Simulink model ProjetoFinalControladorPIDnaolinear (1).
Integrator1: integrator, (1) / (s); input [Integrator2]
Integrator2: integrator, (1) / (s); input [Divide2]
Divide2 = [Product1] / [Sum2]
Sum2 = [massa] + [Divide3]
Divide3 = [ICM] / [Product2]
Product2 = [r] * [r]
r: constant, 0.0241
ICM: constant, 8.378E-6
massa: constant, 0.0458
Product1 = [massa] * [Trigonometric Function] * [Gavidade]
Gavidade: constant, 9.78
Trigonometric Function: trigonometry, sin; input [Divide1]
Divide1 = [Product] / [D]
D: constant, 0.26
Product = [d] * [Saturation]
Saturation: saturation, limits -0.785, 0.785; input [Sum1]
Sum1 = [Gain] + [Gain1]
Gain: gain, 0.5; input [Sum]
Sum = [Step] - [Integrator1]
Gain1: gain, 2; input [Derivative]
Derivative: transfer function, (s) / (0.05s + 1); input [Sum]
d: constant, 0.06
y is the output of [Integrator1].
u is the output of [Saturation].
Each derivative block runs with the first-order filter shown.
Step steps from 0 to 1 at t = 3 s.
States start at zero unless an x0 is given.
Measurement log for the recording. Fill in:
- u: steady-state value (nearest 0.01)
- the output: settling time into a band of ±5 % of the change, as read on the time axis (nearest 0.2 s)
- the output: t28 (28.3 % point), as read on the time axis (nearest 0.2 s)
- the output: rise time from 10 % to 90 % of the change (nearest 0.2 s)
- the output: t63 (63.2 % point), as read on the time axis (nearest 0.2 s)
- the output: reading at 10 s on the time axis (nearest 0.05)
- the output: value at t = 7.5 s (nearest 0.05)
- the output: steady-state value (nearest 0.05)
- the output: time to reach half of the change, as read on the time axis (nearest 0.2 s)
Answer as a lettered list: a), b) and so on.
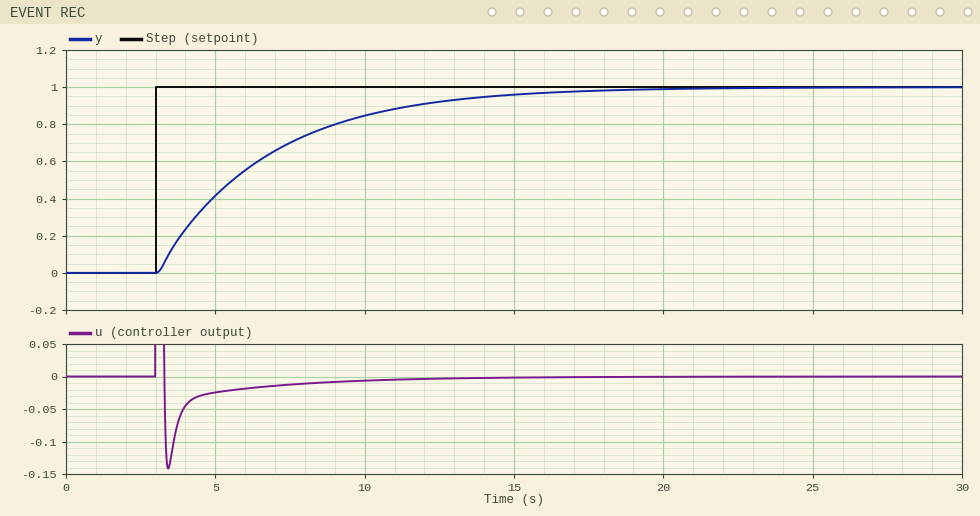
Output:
a) 0.00
b) 14.2 s
c) 4.2 s
d) 8.2 s
e) 6.8 s
f) 0.85
g) 0.70
h) 1.00
i) 5.6 s
